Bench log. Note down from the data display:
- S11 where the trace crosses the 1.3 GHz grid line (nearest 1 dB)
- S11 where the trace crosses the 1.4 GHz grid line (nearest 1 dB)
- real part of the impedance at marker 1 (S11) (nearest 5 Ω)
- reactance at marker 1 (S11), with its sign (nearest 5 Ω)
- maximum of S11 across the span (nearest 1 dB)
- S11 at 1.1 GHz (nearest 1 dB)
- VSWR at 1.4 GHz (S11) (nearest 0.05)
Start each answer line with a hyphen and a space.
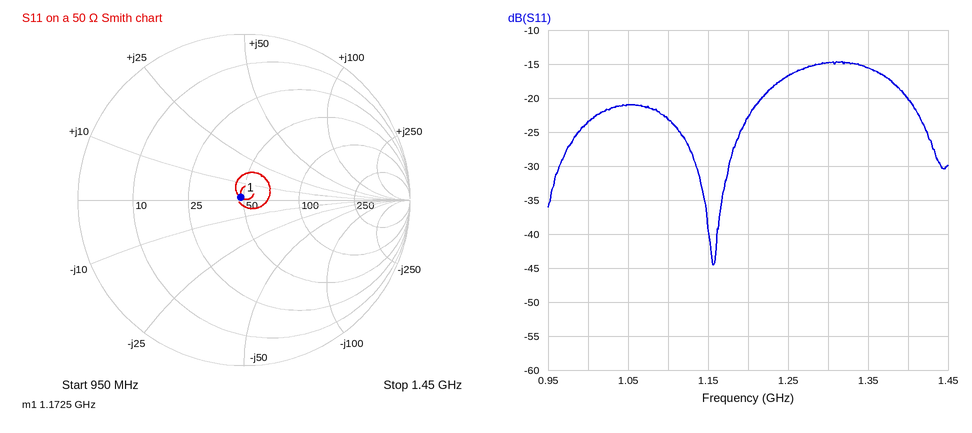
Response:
- -15 dB
- -20 dB
- 50 Ω
- 0 Ω
- -15 dB
- -23 dB
- 1.20
